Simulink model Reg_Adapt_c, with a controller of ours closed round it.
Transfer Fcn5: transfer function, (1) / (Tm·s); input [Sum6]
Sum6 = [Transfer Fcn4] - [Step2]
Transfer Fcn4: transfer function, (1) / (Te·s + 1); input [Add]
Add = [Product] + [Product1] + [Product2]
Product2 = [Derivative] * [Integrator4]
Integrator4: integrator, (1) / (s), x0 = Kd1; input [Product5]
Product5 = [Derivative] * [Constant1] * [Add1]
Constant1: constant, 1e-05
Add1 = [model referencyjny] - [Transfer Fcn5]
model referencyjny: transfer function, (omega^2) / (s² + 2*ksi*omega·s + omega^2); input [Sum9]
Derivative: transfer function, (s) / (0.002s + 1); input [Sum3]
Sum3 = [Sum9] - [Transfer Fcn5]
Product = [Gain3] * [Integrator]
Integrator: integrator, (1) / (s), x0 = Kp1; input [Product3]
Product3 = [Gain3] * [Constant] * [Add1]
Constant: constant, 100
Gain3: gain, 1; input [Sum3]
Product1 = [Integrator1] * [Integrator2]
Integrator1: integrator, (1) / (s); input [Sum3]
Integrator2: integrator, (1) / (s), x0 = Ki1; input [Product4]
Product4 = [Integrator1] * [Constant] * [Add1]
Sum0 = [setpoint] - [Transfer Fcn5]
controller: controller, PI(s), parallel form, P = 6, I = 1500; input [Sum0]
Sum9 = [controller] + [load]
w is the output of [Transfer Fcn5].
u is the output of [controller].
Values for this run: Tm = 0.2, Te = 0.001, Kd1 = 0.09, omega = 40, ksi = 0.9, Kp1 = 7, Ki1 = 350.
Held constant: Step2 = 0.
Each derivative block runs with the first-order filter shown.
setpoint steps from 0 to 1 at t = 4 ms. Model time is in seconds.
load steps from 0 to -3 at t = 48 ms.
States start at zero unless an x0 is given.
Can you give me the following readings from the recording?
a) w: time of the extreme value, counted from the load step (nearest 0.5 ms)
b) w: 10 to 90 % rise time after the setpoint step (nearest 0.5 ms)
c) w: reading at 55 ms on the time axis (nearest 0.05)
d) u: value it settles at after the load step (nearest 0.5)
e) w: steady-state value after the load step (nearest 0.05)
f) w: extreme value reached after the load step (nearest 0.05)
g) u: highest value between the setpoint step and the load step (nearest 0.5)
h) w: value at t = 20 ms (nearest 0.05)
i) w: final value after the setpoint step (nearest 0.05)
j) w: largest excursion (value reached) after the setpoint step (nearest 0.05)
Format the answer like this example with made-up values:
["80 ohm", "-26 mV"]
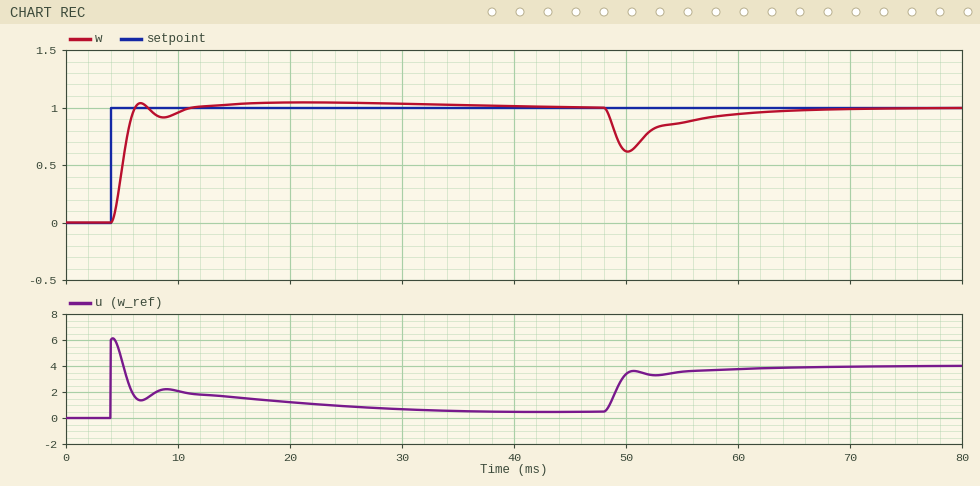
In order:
["2.0 ms", "1.5 ms", "0.85", "4.0", "1.00", "0.60", "6.0", "1.05", "1.00", "1.05"]
